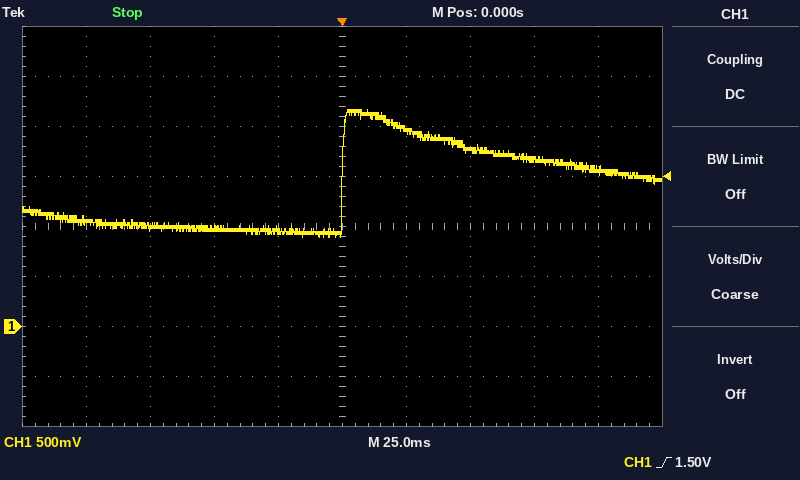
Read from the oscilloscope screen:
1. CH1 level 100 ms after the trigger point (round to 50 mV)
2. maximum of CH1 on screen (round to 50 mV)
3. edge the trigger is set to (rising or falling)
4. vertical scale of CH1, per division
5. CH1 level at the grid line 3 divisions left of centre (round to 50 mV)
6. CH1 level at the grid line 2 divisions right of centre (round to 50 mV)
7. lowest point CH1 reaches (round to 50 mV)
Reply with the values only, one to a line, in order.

1.55 V
2.15 V
rising
500 mV
1.00 V
1.75 V
900 mV
